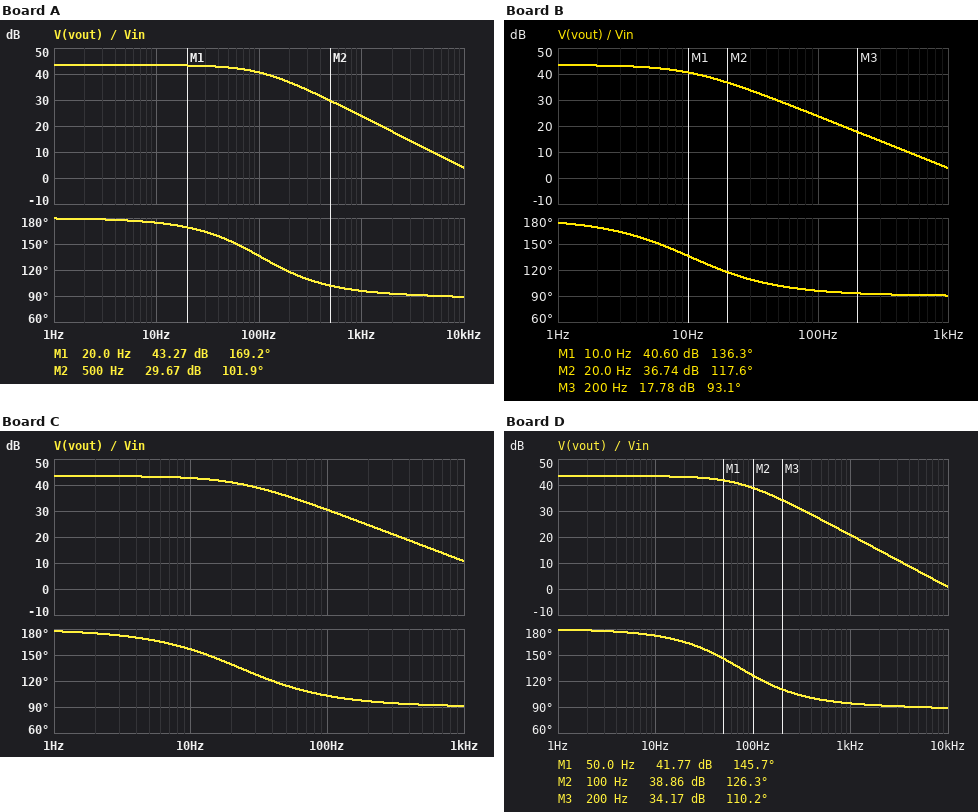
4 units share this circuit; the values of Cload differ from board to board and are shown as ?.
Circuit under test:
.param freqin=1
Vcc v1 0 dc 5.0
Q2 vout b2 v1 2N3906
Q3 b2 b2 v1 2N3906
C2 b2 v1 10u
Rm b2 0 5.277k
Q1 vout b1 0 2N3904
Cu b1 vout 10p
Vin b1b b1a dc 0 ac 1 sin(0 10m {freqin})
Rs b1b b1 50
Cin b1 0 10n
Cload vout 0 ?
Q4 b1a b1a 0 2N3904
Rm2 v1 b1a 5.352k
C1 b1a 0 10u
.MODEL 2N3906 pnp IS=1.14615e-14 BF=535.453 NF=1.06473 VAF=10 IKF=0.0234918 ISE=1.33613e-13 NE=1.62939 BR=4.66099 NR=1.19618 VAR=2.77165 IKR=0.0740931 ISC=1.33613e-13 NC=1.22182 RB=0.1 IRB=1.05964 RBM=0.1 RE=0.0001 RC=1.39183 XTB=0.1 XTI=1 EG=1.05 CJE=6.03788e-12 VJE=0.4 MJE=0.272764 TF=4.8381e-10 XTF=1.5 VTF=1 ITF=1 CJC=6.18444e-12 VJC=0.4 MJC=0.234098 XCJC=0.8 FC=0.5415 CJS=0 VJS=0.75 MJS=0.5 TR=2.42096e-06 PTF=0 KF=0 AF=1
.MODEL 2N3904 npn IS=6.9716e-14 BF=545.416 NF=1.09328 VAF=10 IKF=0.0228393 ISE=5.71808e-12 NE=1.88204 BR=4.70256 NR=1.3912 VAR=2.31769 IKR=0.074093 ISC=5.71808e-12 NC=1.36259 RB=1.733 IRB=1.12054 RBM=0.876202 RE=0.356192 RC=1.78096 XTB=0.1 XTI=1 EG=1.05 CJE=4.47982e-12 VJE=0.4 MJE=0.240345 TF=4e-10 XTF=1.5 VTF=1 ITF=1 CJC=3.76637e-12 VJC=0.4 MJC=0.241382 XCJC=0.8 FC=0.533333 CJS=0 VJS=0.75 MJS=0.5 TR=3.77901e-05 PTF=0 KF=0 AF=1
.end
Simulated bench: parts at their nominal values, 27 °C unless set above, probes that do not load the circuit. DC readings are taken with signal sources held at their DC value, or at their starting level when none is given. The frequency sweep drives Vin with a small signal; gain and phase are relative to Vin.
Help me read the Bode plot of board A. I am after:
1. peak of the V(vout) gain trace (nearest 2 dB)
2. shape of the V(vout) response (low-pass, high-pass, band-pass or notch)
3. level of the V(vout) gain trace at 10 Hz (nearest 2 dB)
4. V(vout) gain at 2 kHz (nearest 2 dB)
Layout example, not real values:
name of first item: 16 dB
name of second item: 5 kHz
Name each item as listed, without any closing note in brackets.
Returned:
peak of the V(vout) gain trace: 44 dB
shape of the V(vout) response: low-pass
level of the V(vout) gain trace at 10 Hz: 44 dB
V(vout) gain at 2 kHz: 18 dB
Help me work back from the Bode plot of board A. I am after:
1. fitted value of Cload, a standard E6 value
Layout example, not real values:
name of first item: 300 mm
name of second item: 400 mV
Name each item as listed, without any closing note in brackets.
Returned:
fitted value of Cload, a standard E6 value: 330 nF
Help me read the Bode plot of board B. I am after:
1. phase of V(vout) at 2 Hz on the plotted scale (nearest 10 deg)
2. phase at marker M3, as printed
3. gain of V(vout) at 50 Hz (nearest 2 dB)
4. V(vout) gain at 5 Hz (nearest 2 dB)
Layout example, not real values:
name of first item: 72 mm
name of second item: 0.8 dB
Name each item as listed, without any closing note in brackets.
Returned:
phase of V(vout) at 2 Hz on the plotted scale: 170 deg
phase at marker M3, as printed: 93.1 deg
gain of V(vout) at 50 Hz: 30 dB
V(vout) gain at 5 Hz: 42 dB
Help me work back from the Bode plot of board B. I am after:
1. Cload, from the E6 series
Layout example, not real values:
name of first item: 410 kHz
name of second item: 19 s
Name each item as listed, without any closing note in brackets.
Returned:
Cload, from the E6 series: 3.3 µF
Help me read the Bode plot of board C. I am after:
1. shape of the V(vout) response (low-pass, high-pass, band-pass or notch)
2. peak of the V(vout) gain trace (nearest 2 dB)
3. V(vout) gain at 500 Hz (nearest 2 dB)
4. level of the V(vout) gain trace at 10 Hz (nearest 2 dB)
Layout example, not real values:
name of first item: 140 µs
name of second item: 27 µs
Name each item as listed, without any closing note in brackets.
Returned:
shape of the V(vout) response: low-pass
peak of the V(vout) gain trace: 44 dB
V(vout) gain at 500 Hz: 16 dB
level of the V(vout) gain trace at 10 Hz: 42 dB
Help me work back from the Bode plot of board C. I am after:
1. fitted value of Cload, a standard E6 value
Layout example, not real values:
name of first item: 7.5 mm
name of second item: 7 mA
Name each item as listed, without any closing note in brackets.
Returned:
fitted value of Cload, a standard E6 value: 1.5 µF
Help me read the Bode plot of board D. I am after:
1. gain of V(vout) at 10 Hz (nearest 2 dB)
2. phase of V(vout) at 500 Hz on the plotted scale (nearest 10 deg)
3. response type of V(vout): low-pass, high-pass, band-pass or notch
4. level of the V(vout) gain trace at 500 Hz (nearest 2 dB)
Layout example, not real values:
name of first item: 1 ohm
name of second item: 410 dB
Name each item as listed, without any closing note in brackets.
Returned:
gain of V(vout) at 10 Hz: 44 dB
phase of V(vout) at 500 Hz on the plotted scale: 100 deg
response type of V(vout): low-pass, high-pass, band-pass or notch: low-pass
level of the V(vout) gain trace at 500 Hz: 26 dB
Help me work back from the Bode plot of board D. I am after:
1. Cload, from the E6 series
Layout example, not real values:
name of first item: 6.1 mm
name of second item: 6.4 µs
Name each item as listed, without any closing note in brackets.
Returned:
Cload, from the E6 series: 470 nF
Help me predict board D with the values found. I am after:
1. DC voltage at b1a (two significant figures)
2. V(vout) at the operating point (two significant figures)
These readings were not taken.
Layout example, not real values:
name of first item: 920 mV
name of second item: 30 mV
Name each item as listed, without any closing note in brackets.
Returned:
DC voltage at b1a: 670 mV
V(vout) at the operating point: 2.6 V
